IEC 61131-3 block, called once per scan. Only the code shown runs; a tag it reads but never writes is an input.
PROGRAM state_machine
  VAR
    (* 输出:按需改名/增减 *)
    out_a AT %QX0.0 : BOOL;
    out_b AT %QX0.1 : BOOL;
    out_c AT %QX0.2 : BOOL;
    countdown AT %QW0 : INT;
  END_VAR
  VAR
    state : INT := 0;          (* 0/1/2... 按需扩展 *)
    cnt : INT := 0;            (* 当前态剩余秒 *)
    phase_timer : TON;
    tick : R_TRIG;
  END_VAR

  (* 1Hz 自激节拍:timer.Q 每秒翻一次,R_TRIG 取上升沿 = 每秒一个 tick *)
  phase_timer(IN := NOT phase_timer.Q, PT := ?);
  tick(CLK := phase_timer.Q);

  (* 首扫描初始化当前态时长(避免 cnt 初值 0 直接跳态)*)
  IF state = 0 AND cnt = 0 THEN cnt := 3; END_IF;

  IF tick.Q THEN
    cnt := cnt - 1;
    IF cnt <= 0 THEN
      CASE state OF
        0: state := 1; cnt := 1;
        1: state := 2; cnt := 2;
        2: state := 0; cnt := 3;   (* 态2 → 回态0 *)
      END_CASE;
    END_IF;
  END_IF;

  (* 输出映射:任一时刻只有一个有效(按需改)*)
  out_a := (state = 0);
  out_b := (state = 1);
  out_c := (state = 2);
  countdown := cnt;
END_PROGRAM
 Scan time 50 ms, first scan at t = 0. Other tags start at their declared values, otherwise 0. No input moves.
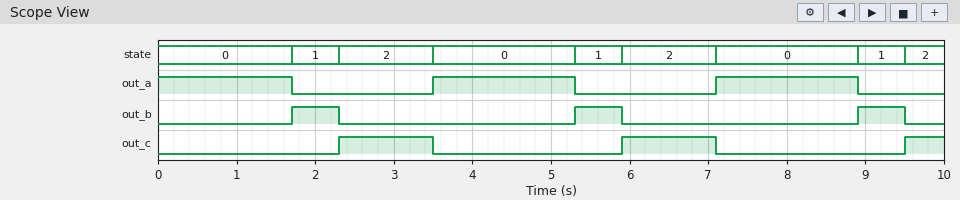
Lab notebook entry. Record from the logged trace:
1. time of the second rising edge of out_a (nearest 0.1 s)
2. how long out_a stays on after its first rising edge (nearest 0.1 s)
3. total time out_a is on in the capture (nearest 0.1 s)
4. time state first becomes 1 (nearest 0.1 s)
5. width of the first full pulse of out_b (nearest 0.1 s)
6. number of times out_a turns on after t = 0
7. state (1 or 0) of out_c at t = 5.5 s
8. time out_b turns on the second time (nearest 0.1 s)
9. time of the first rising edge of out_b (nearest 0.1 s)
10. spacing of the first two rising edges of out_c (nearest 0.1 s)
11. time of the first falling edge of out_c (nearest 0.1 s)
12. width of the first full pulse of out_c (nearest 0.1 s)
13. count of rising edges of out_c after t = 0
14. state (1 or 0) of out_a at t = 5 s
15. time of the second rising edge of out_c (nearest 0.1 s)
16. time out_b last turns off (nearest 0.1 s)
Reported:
7.1 s
1.8 s
5.3 s
1.7 s
0.6 s
2
0
5.3 s
1.7 s
3.6 s
3.5 s
1.2 s
3
1
5.9 s
9.5 s
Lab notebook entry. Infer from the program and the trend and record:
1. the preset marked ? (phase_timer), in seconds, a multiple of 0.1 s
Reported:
0.5 s
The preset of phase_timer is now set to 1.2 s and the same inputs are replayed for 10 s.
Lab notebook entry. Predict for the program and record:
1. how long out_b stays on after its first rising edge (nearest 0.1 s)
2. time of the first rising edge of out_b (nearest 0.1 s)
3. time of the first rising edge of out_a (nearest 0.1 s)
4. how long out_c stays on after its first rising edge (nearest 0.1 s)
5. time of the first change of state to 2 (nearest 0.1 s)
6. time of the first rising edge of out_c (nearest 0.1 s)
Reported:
1.3 s
3.8 s
7.7 s
2.6 s
5.1 s
5.1 s
